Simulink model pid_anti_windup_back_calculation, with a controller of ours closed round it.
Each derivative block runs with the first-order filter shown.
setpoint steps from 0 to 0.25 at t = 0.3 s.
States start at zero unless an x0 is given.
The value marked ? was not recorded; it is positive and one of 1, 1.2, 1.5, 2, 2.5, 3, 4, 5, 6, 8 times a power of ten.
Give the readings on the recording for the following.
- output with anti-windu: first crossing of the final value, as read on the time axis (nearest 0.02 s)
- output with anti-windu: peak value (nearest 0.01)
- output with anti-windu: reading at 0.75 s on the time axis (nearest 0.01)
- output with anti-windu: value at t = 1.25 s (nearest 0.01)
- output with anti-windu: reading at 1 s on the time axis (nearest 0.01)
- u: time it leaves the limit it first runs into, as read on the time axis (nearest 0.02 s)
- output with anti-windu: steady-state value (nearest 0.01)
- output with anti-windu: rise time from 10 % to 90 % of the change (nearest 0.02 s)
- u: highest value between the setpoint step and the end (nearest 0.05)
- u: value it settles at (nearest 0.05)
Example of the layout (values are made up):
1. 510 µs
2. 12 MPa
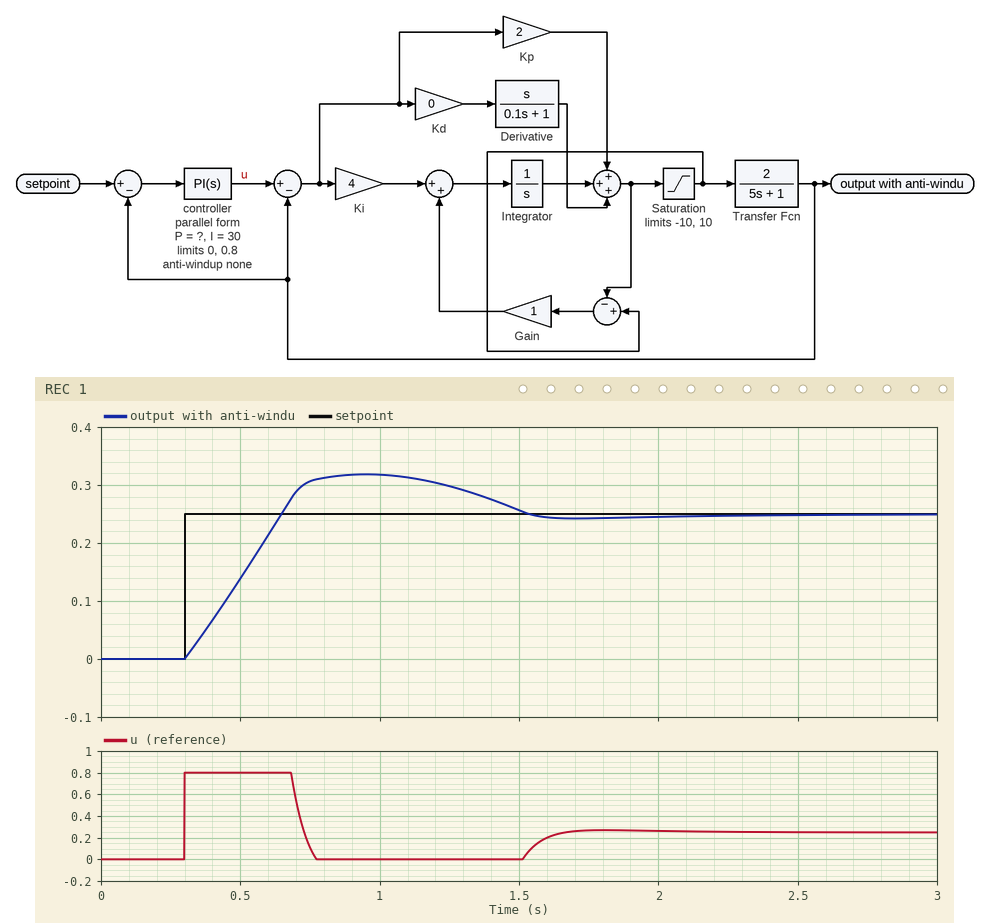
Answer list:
1. 0.64 s
2. 0.32
3. 0.31
4. 0.30
5. 0.32
6. 0.68 s
7. 0.25
8. 0.28 s
9. 0.80
10. 0.25
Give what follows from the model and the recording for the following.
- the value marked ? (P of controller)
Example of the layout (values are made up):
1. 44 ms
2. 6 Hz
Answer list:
1. 20
